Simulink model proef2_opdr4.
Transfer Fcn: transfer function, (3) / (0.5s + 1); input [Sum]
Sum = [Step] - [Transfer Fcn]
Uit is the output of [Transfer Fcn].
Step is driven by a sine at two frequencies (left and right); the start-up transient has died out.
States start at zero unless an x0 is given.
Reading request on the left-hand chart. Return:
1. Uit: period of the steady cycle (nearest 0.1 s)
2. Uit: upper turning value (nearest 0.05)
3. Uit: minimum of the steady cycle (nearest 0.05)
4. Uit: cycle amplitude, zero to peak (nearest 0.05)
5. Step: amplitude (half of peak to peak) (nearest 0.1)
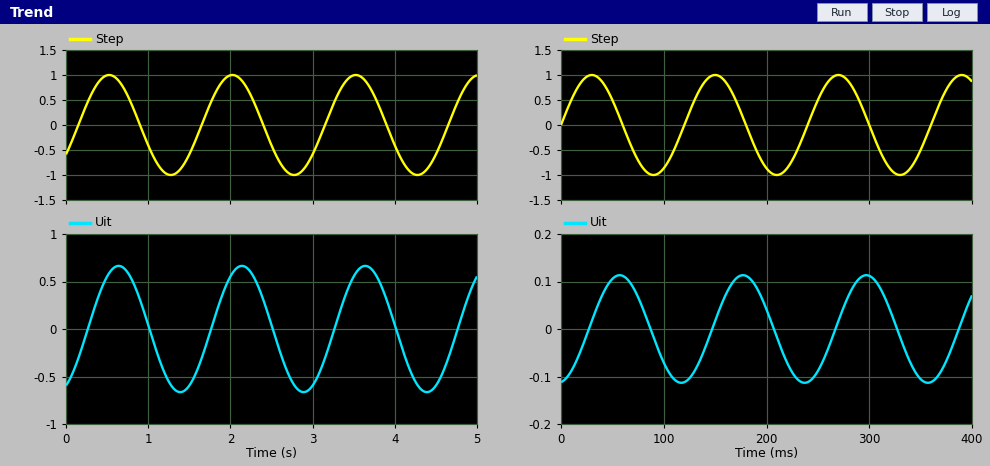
1.5 s
0.65
-0.65
0.65
1.0
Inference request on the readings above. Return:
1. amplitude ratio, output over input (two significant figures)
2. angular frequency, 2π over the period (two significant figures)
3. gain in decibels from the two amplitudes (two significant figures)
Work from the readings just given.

0.65
4.2 rad/s
-3.7 dB
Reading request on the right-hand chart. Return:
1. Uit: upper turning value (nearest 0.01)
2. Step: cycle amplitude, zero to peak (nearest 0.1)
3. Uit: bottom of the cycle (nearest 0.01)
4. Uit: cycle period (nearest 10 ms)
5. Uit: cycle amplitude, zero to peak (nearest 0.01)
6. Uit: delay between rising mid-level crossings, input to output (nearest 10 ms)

0.11
1.0
-0.11
120 ms
0.11
30 ms
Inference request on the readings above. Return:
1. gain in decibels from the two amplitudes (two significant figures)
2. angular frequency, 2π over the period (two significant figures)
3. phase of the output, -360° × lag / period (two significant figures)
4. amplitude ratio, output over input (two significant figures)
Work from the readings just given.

-19 dB
0.052 rad/ms
-90°
0.11
